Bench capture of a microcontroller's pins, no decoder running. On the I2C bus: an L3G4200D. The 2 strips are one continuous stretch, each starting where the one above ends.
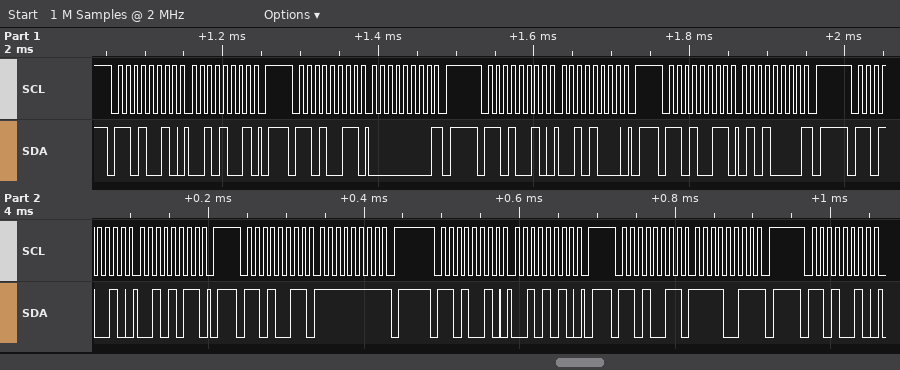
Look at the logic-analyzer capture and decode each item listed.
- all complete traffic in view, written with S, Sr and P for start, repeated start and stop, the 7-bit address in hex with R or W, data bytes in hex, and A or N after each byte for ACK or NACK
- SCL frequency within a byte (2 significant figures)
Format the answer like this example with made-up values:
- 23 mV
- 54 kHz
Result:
- S 69W A 29 A P S 69R A 00 N P S 69W A 28 A P S 69R A 50 N P S 69W A 2B A P S 69R A FF N P S 69W A 2A A P S 69R A F3 N P S 69W A
- 100 kHz
